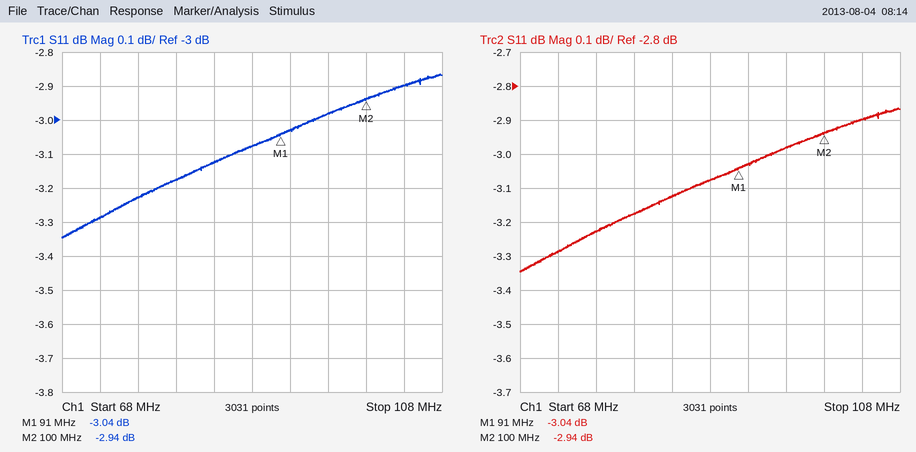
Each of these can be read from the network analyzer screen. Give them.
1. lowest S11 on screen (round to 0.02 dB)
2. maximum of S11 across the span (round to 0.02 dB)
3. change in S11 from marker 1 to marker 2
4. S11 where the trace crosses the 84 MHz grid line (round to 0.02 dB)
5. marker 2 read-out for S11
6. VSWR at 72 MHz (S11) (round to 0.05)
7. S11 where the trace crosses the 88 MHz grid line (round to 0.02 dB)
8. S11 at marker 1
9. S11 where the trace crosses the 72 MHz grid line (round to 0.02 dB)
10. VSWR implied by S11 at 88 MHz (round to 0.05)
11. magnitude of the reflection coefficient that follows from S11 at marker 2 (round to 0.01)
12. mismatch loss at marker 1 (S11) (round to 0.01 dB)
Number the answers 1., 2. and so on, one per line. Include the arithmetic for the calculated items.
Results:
1. -3.34 dB
2. -2.86 dB
3. -2.94 − (-3.04) = 0.10 dB
4. -3.12 dB
5. -2.94 dB
6. |Γ| = 10^(-3.28/20) = 0.6855; VSWR = (1 + 0.6855)/(1 − 0.6855) ≈ 5.36, so 5.35 to the nearest 0.05
7. -3.08 dB
8. -3.04 dB
9. -3.28 dB
10. |Γ| = 10^(-3.08/20) = 0.7015; VSWR = (1 + 0.7015)/(1 − 0.7015) ≈ 5.70
11. 10^(-2.94/20) ≈ 0.71
12. −10 log10(1 − 10^(-3.04/10)) ≈ 2.98 dB
